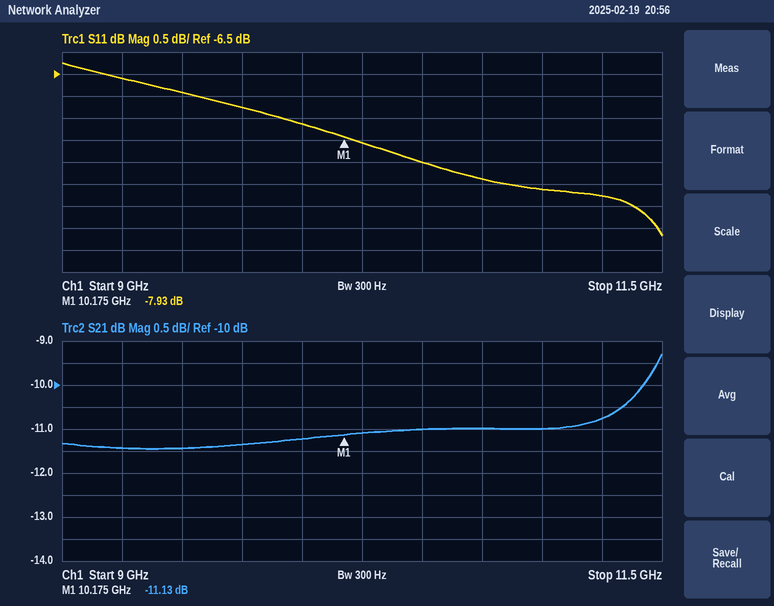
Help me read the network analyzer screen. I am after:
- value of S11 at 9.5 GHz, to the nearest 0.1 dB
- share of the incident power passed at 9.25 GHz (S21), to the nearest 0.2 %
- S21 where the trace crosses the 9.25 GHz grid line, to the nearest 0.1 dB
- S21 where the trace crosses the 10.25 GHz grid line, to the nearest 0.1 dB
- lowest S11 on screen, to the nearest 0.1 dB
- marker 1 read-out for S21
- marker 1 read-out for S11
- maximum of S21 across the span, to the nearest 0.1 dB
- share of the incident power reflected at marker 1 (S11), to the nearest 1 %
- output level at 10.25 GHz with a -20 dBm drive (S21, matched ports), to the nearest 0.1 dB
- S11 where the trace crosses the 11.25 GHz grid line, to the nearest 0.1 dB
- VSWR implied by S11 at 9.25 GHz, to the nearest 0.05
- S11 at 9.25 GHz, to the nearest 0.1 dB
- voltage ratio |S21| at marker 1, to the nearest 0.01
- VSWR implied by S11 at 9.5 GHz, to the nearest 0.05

-6.9 dB
7.2 %
-11.4 dB
-11.1 dB
-10.2 dB
-11.13 dB
-7.93 dB
-9.3 dB
16 %
-31.1 dBm
-9.3 dB
2.75
-6.6 dB
0.28
2.65
